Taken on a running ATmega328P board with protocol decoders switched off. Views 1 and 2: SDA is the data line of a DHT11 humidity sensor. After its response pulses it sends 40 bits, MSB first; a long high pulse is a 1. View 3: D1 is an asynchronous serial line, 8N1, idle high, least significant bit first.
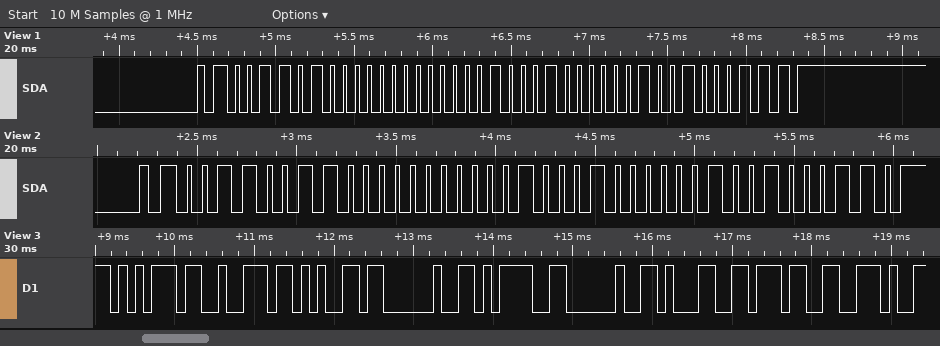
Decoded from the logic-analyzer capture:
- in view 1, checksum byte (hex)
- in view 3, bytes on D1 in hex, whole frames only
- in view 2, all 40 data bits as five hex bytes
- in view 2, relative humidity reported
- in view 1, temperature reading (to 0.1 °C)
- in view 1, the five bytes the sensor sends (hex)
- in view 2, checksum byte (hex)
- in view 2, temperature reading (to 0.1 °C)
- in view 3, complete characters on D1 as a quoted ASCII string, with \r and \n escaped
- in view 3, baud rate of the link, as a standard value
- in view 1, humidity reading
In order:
0x47
75 72 65 20 3D 20 31 37 2E
33 00 11 02 46
51 %
17.2 °C
34 00 11 02 47
0x46
17.2 °C
"ure = 17."
9600 baud
52 %
